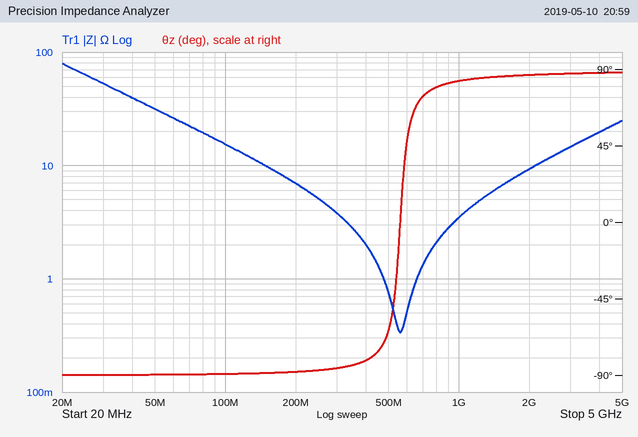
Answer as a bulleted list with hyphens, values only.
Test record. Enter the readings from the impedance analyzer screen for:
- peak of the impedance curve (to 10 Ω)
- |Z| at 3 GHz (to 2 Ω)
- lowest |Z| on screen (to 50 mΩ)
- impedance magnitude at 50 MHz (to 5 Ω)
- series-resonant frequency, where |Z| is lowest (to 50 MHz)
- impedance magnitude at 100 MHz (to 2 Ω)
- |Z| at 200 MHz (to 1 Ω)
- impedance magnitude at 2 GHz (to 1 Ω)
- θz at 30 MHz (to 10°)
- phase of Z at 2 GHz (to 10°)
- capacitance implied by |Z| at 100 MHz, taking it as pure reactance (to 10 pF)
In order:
- 80 Ω
- 14 Ω
- 350 mΩ
- 30 Ω
- 550 MHz
- 16 Ω
- 7 Ω
- 9 Ω
- -90°
- 90°
- 100 pF
